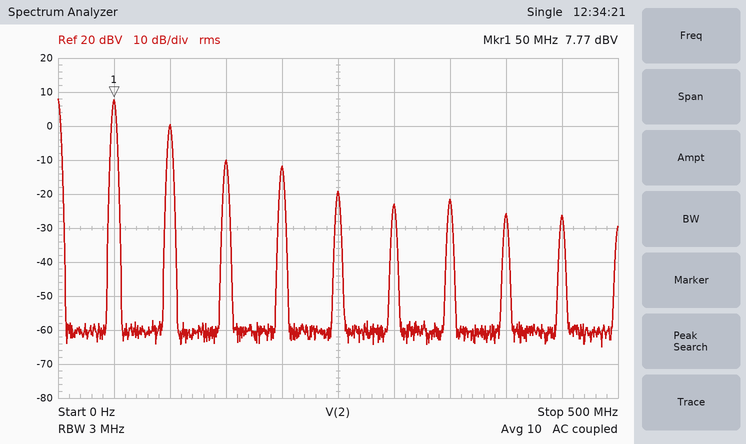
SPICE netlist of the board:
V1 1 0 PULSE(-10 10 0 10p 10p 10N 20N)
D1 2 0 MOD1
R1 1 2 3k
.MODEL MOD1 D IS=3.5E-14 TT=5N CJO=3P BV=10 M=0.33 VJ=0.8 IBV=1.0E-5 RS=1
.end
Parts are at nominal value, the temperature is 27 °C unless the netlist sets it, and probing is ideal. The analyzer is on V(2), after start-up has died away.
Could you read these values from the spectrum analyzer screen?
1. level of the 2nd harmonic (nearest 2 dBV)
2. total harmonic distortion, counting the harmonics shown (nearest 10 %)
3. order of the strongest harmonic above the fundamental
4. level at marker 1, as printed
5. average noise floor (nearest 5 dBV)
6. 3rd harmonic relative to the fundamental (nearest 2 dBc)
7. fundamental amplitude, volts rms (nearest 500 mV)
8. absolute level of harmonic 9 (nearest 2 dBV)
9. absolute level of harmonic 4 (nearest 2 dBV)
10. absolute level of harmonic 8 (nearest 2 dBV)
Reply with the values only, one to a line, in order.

0 dBV
50 %
2
7.77 dBV
-60 dBV
-18 dBc
2.5 V
-26 dBV
-12 dBV
-26 dBV
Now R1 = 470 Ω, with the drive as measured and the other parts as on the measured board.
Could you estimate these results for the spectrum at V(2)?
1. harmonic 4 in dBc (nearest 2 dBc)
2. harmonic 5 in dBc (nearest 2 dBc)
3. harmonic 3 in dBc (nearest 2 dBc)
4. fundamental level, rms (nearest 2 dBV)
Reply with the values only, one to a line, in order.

-14 dBc
-16 dBc
-30 dBc
12 dBV
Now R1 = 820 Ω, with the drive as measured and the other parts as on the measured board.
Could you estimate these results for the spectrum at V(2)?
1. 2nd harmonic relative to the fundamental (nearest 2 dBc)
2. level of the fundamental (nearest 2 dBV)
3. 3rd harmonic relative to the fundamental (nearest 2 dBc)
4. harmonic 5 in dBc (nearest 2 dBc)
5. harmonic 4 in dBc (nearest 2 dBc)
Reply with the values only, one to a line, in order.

-6 dBc
12 dBV
-22 dBc
-18 dBc
-14 dBc
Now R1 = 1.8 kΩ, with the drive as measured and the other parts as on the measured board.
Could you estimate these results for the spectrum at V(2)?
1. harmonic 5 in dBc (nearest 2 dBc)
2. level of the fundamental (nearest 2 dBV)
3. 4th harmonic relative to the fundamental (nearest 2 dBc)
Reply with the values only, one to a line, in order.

-22 dBc
10 dBV
-16 dBc
